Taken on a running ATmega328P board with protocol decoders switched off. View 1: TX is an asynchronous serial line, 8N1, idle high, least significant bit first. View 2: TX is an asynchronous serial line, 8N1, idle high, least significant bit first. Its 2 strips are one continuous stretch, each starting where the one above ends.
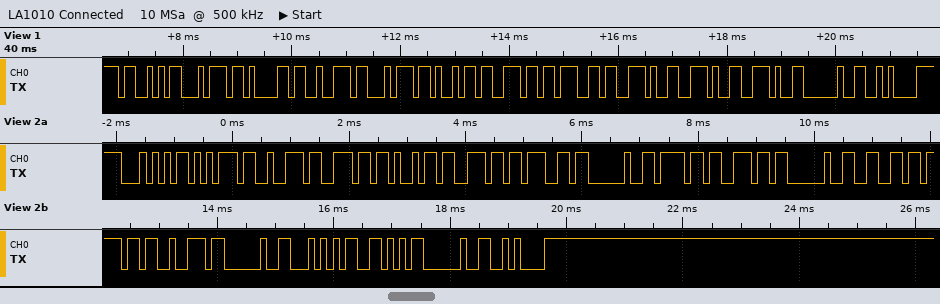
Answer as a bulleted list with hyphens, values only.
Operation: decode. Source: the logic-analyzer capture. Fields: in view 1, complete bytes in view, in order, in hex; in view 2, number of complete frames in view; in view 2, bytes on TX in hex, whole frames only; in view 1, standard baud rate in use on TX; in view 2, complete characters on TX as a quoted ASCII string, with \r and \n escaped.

- 0x53 0x74 0x61 0x72 0x74 0x69 0x6E 0x67 0x2E 0x2E 0x2E 0x20 0x0A
- 19
- 54 75 72 6E 69 6E 67 20 6F 6E 20 66 6F 72 20 54 56 20 0A
- 9600 baud
- "Turning on for TV \n"
